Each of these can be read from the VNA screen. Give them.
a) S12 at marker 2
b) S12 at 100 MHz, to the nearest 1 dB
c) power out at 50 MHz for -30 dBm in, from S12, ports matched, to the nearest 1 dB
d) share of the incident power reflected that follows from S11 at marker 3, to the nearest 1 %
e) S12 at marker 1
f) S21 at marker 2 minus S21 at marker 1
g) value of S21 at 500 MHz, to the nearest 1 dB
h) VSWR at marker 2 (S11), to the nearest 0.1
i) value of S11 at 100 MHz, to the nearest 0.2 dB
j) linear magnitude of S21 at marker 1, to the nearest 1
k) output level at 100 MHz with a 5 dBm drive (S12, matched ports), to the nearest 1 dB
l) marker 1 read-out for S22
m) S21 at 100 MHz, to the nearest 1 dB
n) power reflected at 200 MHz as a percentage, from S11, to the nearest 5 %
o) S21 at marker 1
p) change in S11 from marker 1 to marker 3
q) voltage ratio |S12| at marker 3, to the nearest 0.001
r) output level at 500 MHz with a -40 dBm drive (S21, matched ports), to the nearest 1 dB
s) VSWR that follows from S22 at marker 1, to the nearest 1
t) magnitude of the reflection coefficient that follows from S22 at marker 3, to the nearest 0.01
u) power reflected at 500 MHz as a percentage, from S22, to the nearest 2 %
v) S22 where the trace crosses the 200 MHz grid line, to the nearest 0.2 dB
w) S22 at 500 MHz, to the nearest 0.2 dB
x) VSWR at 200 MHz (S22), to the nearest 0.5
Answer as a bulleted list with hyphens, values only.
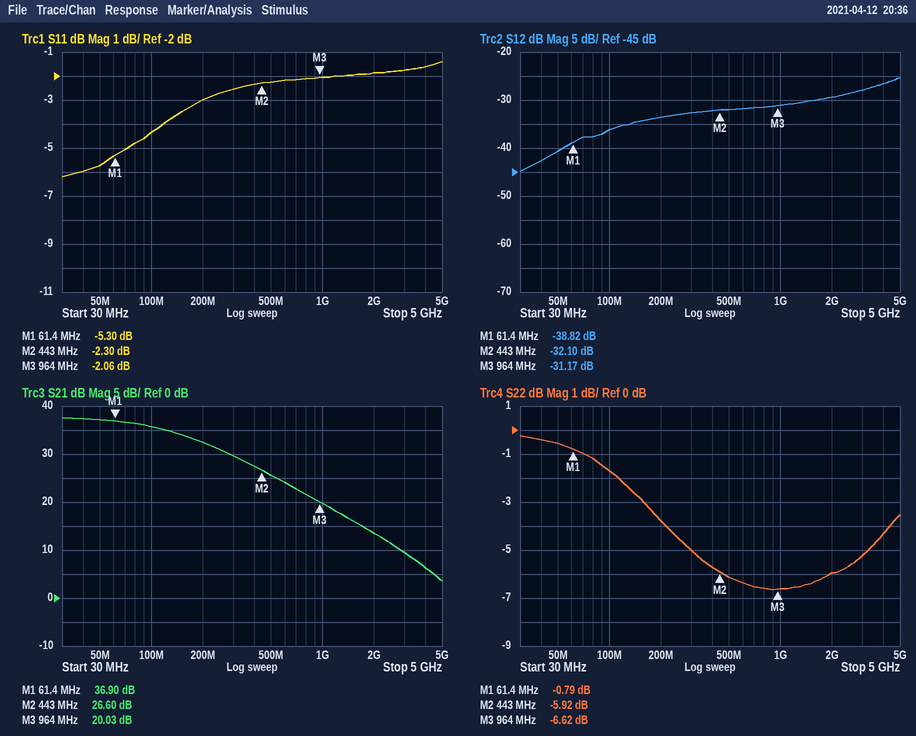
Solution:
- -32.10 dB
- -36 dB
- -71 dBm
- 62 %
- -38.82 dB
- -10.30 dB
- 26 dB
- 7.6
- -4.4 dB
- 70
- -31 dBm
- -0.79 dB
- 36 dB
- 50 %
- 36.90 dB
- 3.24 dB
- 0.028
- -14 dBm
- 22
- 0.47
- 24 %
- -3.8 dB
- -6.2 dB
- 4.5
